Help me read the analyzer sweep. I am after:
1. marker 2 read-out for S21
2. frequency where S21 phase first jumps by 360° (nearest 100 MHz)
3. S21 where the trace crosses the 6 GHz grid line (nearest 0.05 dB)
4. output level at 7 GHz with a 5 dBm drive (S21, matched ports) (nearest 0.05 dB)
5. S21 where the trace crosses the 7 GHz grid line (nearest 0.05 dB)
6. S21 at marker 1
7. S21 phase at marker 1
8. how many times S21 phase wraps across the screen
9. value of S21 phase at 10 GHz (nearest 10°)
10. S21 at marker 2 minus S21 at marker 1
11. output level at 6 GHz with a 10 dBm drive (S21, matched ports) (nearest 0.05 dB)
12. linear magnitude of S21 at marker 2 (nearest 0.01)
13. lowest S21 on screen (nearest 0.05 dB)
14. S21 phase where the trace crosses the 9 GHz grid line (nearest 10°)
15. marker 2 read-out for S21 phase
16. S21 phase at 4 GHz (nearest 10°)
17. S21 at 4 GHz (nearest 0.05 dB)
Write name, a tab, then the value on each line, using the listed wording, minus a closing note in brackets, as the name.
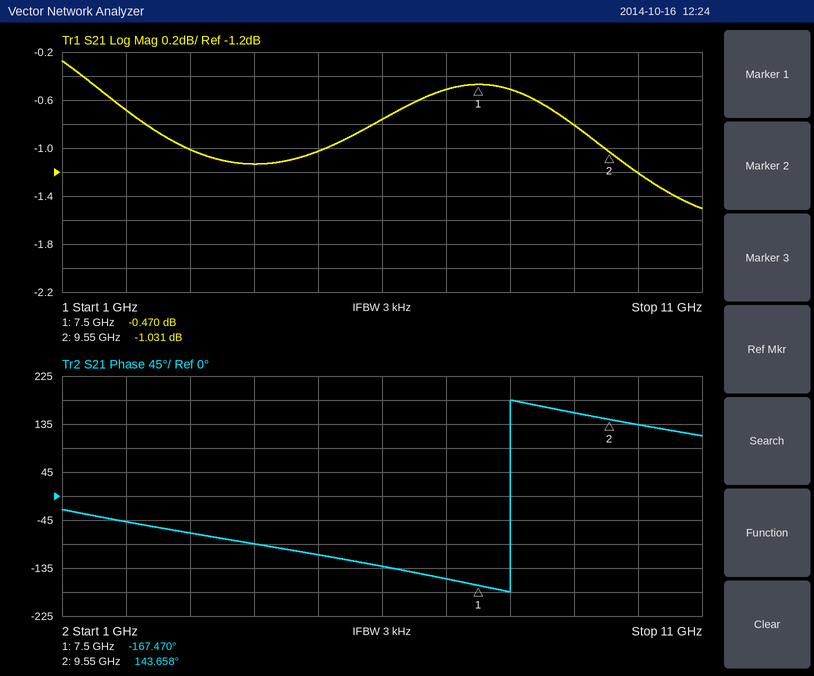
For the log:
marker 2 read-out for S21	-1.031 dB
frequency where S21 phase first jumps by 360°	8.0 GHz
S21 where the trace crosses the 6 GHz grid line	-0.75 dB
output level at 7 GHz with a 5 dBm drive (S21, matched ports)	4.50 dBm
S21 where the trace crosses the 7 GHz grid line	-0.50 dB
S21 at marker 1	-0.470 dB
S21 phase at marker 1	-167.470°
how many times S21 phase wraps across the screen	1
value of S21 phase at 10 GHz	130°
S21 at marker 2 minus S21 at marker 1	-0.561 dB
output level at 6 GHz with a 10 dBm drive (S21, matched ports)	9.25 dBm
linear magnitude of S21 at marker 2	0.89
lowest S21 on screen	-1.50 dB
S21 phase where the trace crosses the 9 GHz grid line	160°
marker 2 read-out for S21 phase	143.658°
S21 phase at 4 GHz	-90°
S21 at 4 GHz	-1.15 dB
